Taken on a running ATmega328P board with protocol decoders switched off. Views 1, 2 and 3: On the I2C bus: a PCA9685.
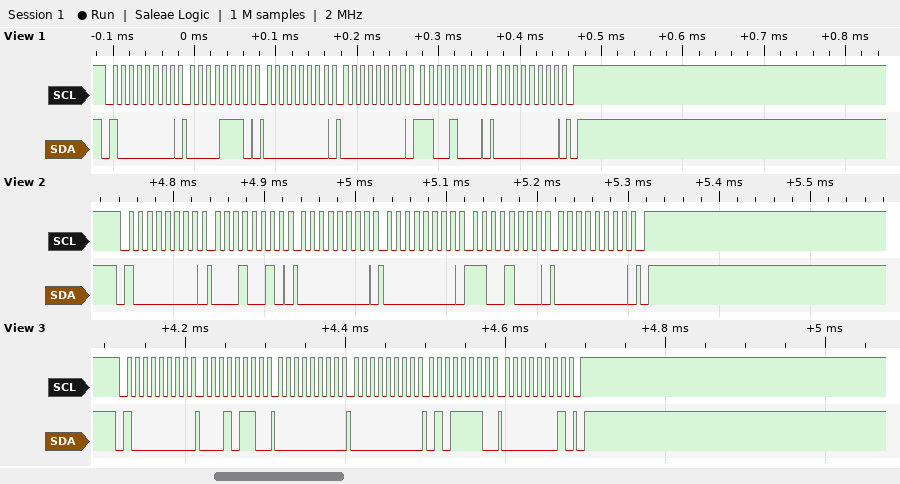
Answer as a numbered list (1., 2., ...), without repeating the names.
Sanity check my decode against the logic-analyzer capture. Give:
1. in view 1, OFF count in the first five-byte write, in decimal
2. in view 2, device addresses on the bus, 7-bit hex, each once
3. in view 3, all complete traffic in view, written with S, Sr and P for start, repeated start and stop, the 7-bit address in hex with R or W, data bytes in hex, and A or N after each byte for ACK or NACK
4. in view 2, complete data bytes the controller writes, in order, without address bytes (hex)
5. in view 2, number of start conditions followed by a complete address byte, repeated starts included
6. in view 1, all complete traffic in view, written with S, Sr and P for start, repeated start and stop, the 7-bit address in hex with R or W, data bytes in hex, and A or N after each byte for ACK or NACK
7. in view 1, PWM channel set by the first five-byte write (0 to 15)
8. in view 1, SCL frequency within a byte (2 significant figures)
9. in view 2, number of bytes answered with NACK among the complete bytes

1. 200
2. 0x40
3. S 40W A 16 A 00 A 00 A 5E A 01 A P
4. 12 00 00 C8 00
5. 1
6. S 40W A 0E A 00 A 00 A C8 A 00 A P
7. 2
8. 100 kHz
9. 0
